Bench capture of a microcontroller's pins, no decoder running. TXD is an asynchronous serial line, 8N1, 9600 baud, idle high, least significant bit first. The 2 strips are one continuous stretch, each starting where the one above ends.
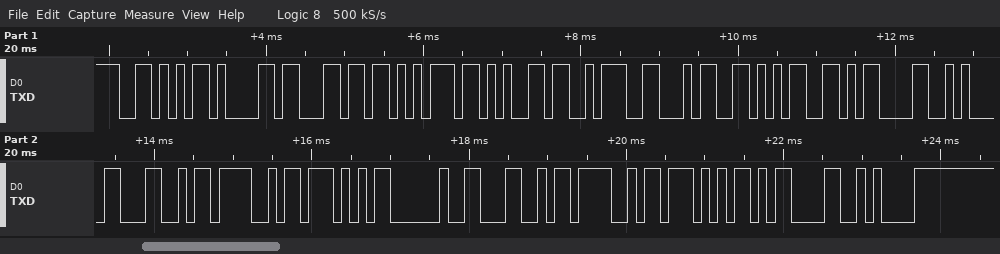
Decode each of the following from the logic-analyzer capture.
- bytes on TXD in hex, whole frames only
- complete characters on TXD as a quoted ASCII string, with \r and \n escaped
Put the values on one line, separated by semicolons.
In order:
56 61 6C 75 65 3A 34 35 0D 0A 4C 4F 57 20 4C 4F 57 0D 0A; "Value:45\r\nLOW LOW\r\n"
